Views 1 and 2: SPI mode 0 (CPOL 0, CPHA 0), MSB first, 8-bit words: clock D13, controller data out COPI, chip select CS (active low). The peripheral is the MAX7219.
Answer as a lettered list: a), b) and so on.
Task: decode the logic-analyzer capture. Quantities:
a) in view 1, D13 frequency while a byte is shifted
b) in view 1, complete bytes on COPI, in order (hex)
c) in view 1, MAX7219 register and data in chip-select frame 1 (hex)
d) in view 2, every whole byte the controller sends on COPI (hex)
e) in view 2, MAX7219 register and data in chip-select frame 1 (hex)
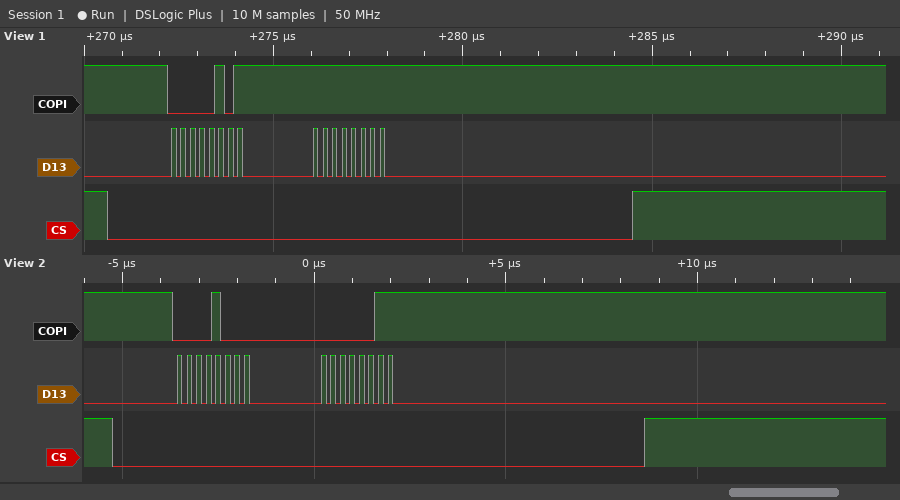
a) 4 MHz
b) 05 FF
c) register 0x5, data 0xFF
d) 08 03
e) register 0x8, data 0x03
